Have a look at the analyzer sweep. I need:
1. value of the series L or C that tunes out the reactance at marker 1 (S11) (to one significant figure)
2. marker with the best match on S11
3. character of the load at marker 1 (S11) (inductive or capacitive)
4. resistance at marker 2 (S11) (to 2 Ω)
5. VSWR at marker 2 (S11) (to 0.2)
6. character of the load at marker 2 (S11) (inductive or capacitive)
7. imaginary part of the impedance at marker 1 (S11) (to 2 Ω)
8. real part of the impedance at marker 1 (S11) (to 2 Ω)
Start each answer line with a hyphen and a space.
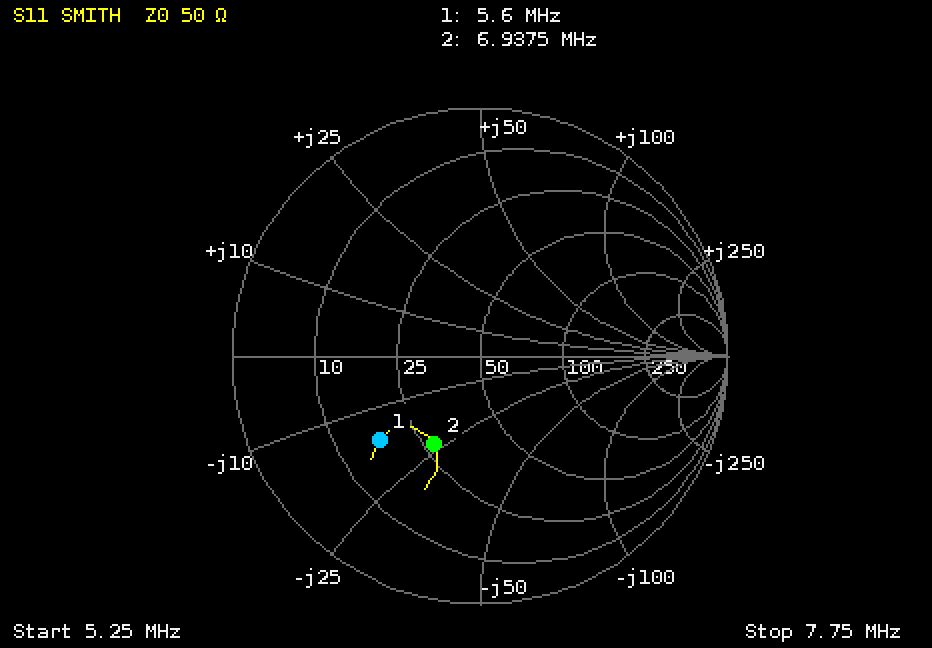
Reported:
- 500 nH
- marker 2
- capacitive
- 28 Ω
- 2.4
- capacitive
- -16 Ω
- 18 Ω
